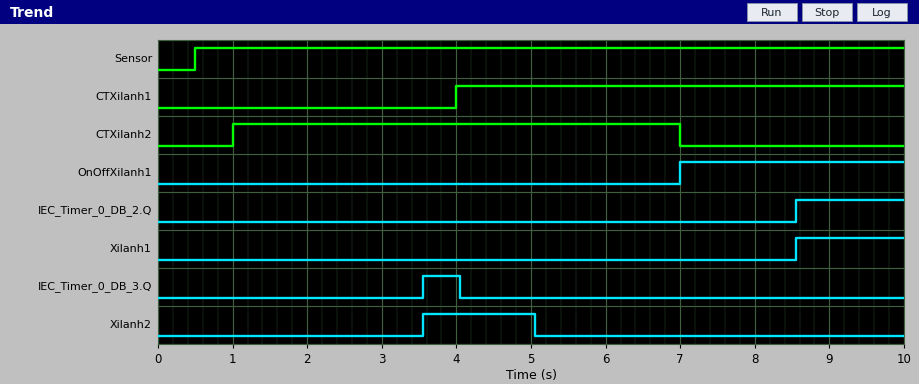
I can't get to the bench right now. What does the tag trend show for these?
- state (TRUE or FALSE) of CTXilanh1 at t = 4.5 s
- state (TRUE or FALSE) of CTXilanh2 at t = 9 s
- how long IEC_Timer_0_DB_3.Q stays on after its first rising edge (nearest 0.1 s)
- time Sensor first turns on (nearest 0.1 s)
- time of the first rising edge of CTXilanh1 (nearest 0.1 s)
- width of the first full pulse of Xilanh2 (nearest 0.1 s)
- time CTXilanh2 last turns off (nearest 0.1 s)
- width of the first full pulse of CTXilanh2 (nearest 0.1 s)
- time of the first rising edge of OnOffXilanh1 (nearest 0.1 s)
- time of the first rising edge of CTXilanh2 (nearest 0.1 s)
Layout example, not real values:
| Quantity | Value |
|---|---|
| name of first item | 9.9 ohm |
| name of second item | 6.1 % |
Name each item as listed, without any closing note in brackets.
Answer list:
| Quantity | Value |
|---|---|
| state (TRUE or FALSE) of CTXilanh1 at t = 4.5 s | TRUE |
| state (TRUE or FALSE) of CTXilanh2 at t = 9 s | FALSE |
| how long IEC_Timer_0_DB_3.Q stays on after its first rising edge | 0.5 s |
| time Sensor first turns on | 0.5 s |
| time of the first rising edge of CTXilanh1 | 4.0 s |
| width of the first full pulse of Xilanh2 | 1.5 s |
| time CTXilanh2 last turns off | 7.0 s |
| width of the first full pulse of CTXilanh2 | 6.0 s |
| time of the first rising edge of OnOffXilanh1 | 7.0 s |
| time of the first rising edge of CTXilanh2 | 1.0 s |
